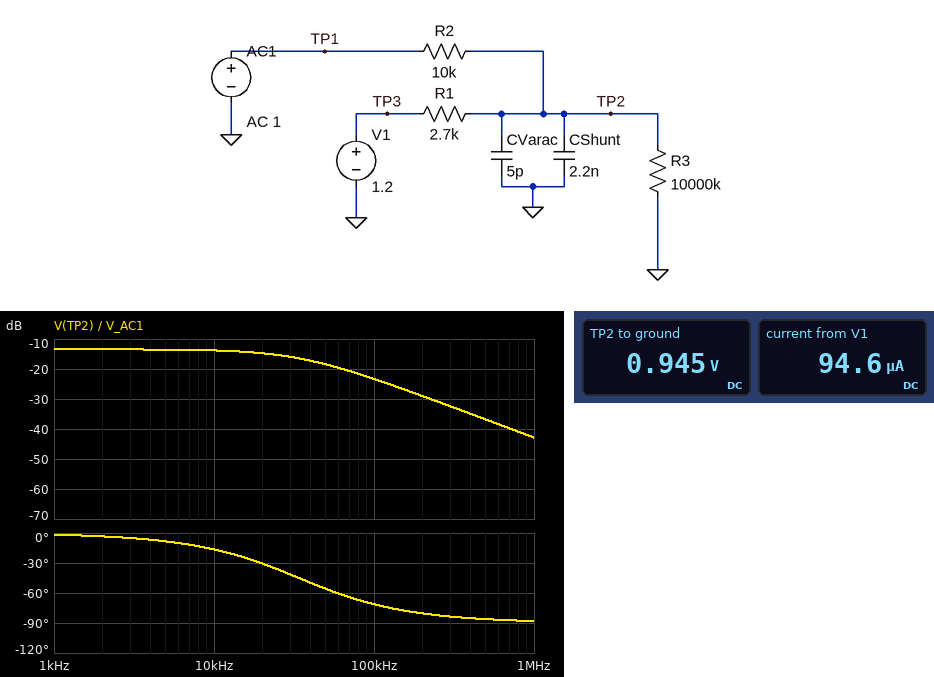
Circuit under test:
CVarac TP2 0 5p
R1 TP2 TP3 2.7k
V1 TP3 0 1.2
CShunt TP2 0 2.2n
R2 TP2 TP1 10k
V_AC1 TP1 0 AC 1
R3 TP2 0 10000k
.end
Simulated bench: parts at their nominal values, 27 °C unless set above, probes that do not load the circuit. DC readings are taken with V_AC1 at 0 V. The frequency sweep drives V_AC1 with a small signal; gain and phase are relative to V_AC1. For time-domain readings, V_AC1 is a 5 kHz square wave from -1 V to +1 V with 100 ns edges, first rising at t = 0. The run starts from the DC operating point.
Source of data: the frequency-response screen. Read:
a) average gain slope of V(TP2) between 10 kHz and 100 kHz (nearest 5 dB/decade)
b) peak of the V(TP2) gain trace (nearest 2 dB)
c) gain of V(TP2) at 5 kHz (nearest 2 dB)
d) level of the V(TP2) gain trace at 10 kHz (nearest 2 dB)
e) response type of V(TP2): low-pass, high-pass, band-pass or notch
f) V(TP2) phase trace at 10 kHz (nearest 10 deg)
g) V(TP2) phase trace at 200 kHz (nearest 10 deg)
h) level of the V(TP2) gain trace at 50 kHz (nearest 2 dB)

-10 dB/decade
-14 dB
-14 dB
-14 dB
low-pass
-20 deg
-80 deg
-18 dB
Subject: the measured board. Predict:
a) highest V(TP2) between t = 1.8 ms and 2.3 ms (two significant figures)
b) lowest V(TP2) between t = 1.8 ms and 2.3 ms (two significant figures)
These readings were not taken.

1.2 V
730 mV
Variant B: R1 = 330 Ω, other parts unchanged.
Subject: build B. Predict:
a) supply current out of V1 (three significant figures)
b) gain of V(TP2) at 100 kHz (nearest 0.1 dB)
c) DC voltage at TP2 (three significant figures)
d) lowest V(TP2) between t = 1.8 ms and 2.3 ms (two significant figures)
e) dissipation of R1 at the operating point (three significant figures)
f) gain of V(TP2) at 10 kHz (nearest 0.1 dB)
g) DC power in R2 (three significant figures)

116 µA
-30.7 dB
1.16 V
1.1 V
4.46 µW
-29.9 dB
135 µW
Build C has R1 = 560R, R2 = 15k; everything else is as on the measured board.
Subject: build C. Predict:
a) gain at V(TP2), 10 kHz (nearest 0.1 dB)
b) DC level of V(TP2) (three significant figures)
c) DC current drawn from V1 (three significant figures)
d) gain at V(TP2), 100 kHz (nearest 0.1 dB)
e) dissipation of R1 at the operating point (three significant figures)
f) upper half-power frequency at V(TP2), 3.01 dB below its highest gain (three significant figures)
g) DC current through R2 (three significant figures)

-28.9 dB
1.16 V
77.2 µA
-30.8 dB
3.34 µW
134 kHz
77.1 µA
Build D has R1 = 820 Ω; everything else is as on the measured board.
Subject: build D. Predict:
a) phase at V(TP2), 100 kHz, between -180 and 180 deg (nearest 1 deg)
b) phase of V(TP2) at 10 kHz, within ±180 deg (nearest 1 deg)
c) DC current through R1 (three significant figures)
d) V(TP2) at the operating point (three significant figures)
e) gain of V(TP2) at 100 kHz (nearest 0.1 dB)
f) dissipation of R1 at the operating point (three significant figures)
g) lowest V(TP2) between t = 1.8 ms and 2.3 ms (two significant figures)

-46 deg
-6 deg
111 µA
1.11 V
-25.6 dB
10.1 µW
1.0 V
